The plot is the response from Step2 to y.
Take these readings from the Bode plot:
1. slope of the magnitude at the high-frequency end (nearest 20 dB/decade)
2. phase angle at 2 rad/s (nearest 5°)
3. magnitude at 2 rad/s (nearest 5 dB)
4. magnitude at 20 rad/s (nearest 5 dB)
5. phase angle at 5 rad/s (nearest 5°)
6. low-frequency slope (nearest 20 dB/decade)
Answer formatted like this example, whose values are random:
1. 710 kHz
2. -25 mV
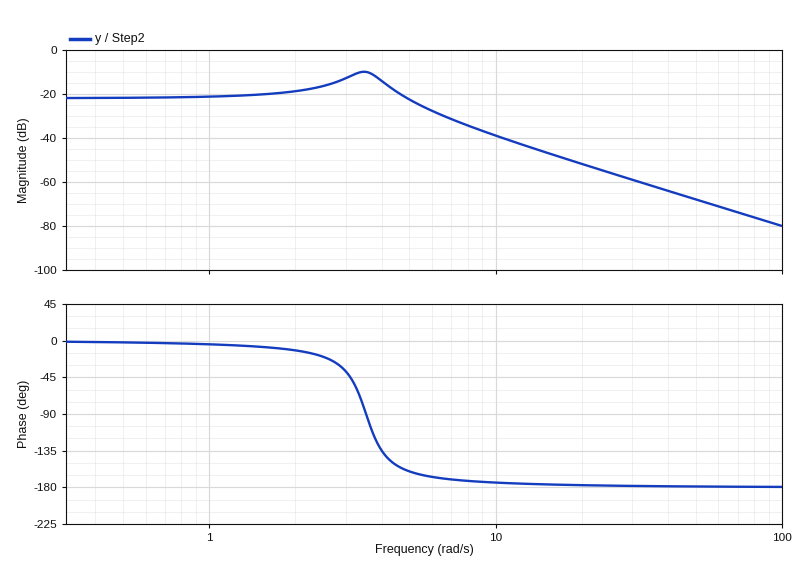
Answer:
1. -40 dB/decade
2. -10°
3. -20 dB
4. -50 dB
5. -160°
6. 0 dB/decade
